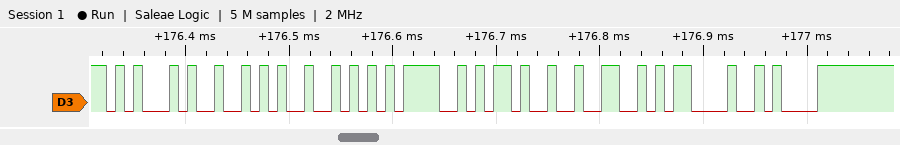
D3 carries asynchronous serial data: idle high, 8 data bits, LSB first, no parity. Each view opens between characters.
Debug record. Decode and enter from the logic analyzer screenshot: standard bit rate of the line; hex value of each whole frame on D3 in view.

115200 baud
45, 52, 52, 3D, 2D, 32, 0D, 0A
